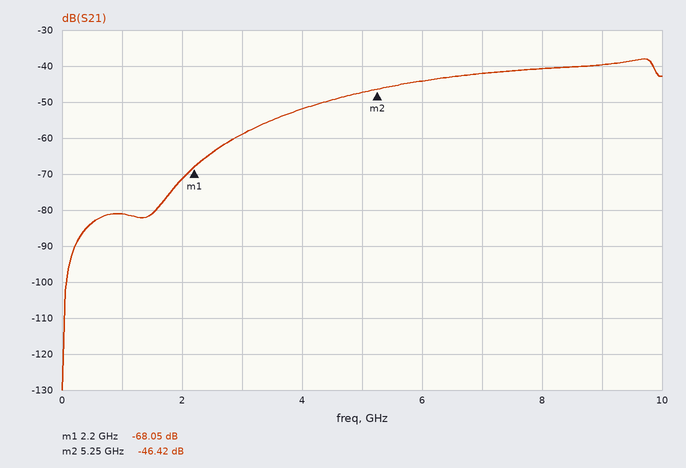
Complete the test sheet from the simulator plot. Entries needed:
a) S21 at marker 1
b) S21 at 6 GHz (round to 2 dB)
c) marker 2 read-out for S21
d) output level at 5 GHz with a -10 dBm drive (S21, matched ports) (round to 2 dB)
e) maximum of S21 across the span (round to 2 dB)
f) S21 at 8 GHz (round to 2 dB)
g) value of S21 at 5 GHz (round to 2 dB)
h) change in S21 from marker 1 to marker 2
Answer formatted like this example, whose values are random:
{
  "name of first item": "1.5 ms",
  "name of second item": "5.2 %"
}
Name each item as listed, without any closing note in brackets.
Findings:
{
  "S21 at marker 1": "-68.05 dB",
  "S21 at 6 GHz": "-44 dB",
  "marker 2 read-out for S21": "-46.42 dB",
  "output level at 5 GHz with a -10 dBm drive (S21, matched ports)": "-58 dBm",
  "maximum of S21 across the span": "-38 dB",
  "S21 at 8 GHz": "-40 dB",
  "value of S21 at 5 GHz": "-48 dB",
  "change in S21 from marker 1 to marker 2": "21.63 dB"
}
